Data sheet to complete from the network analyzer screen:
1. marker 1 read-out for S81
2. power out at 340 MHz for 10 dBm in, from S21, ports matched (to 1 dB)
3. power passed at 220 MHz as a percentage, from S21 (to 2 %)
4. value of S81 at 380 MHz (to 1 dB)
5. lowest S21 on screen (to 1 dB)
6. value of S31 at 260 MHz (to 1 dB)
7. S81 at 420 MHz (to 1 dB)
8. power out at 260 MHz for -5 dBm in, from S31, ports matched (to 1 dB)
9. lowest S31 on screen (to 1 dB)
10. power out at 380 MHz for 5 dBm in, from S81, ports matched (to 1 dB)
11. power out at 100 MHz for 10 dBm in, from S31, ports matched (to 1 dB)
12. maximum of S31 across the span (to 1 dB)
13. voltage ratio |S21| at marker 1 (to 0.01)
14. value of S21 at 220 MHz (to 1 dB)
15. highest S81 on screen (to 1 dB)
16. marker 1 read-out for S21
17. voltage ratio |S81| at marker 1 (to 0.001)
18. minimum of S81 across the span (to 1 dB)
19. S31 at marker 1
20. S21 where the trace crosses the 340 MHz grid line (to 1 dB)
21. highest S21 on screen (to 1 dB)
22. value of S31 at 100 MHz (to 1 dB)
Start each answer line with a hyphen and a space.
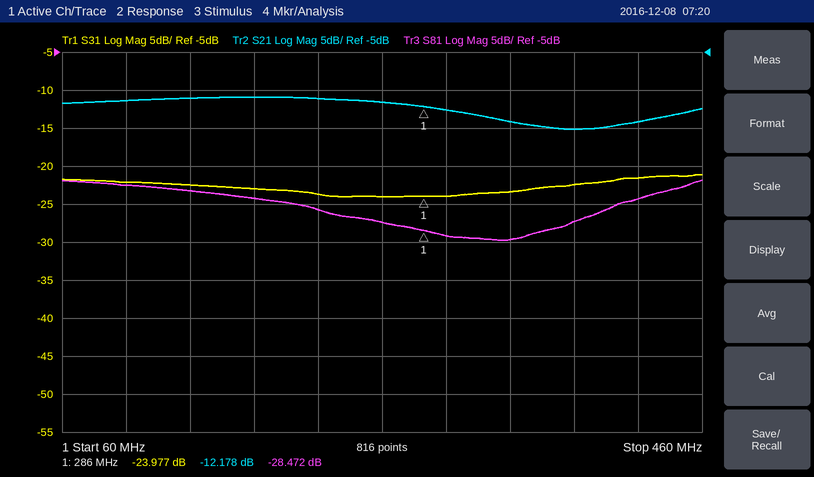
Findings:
- -28.472 dB
- -4 dBm
- 8 %
- -27 dB
- -15 dB
- -24 dB
- -24 dB
- -29 dBm
- -24 dB
- -22 dBm
- -12 dBm
- -21 dB
- 0.25
- -11 dB
- -22 dB
- -12.178 dB
- 0.038
- -30 dB
- -23.977 dB
- -14 dB
- -11 dB
- -22 dB
